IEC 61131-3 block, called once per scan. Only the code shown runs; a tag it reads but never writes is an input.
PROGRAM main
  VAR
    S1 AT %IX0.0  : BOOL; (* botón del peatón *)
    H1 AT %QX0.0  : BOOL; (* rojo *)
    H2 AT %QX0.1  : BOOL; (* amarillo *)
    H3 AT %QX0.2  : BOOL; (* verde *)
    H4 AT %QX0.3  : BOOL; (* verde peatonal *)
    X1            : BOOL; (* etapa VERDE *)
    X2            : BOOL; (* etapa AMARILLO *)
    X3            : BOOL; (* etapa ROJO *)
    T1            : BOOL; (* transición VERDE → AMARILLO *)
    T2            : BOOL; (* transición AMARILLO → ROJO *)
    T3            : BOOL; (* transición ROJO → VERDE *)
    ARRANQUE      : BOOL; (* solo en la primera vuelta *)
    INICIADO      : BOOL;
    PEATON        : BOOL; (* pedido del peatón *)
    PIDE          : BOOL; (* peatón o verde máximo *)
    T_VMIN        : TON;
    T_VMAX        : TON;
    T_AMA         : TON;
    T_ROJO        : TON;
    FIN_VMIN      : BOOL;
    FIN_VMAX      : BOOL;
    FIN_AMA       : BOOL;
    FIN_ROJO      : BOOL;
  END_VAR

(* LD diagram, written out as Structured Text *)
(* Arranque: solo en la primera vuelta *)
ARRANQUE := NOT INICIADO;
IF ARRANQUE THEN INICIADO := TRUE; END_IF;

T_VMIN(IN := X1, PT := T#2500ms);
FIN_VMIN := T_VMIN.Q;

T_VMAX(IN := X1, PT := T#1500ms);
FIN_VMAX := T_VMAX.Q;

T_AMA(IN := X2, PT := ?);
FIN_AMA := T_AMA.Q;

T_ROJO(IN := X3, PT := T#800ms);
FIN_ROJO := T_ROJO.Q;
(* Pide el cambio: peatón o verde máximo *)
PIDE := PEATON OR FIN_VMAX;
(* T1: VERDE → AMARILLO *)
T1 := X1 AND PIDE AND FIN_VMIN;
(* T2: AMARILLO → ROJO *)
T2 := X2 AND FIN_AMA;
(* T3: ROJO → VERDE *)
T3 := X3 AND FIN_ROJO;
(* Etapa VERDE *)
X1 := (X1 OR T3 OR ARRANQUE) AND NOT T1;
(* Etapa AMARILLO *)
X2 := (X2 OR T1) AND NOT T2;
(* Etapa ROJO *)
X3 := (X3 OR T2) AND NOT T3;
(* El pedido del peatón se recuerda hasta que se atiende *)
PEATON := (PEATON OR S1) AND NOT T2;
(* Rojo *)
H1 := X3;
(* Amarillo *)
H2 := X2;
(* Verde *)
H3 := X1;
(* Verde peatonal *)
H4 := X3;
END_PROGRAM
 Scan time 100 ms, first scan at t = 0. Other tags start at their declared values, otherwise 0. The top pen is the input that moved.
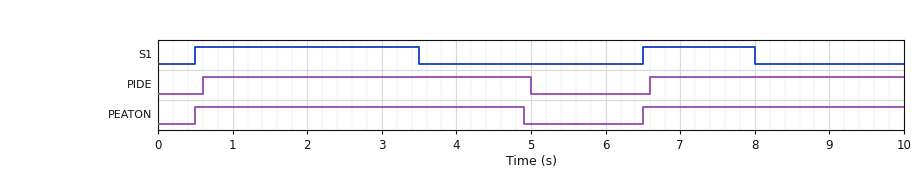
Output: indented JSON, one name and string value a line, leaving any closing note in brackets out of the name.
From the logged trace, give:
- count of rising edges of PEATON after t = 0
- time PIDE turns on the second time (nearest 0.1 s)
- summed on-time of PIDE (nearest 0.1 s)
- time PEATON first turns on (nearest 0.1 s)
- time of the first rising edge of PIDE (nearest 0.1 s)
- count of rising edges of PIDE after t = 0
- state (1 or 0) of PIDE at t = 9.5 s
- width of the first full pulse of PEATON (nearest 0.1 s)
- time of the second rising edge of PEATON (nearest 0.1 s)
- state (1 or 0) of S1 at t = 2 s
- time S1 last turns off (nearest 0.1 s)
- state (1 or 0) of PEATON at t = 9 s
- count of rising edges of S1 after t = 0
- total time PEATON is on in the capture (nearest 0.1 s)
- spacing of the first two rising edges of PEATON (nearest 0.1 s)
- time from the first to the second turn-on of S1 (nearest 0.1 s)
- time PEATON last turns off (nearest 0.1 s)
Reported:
{
  "count of rising edges of PEATON after t = 0": "2",
  "time PIDE turns on the second time": "6.6 s",
  "summed on-time of PIDE": "7.8 s",
  "time PEATON first turns on": "0.5 s",
  "time of the first rising edge of PIDE": "0.6 s",
  "count of rising edges of PIDE after t = 0": "2",
  "state (1 or 0) of PIDE at t = 9.5 s": "1",
  "width of the first full pulse of PEATON": "4.4 s",
  "time of the second rising edge of PEATON": "6.5 s",
  "state (1 or 0) of S1 at t = 2 s": "1",
  "time S1 last turns off": "8.0 s",
  "state (1 or 0) of PEATON at t = 9 s": "1",
  "count of rising edges of S1 after t = 0": "2",
  "total time PEATON is on in the capture": "7.9 s",
  "spacing of the first two rising edges of PEATON": "6.0 s",
  "time from the first to the second turn-on of S1": "6.0 s",
  "time PEATON last turns off": "4.9 s"
}
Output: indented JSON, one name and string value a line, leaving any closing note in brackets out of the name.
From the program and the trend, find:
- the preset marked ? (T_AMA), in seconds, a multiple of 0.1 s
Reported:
{
  "the preset marked ? (T_AMA), in seconds, a multiple of 0.1 s": "2.2 s"
}
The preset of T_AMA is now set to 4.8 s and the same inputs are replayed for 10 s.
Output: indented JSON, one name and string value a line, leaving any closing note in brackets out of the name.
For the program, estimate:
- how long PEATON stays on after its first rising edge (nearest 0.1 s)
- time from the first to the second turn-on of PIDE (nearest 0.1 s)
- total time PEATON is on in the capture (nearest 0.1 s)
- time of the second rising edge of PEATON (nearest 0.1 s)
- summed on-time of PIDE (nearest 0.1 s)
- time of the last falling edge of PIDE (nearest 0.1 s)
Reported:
{
  "how long PEATON stays on after its first rising edge": "7.0 s",
  "time from the first to the second turn-on of PIDE": "7.1 s",
  "total time PEATON is on in the capture": "9.4 s",
  "time of the second rising edge of PEATON": "7.6 s",
  "summed on-time of PIDE": "9.3 s",
  "time of the last falling edge of PIDE": "7.6 s"
}
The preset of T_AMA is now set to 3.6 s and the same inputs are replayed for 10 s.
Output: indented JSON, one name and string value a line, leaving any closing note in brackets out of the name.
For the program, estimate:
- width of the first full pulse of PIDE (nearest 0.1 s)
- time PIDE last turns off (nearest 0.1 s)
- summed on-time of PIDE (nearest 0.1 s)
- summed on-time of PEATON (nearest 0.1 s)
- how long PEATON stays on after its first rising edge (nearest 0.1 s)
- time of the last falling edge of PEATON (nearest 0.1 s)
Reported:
{
  "width of the first full pulse of PIDE": "5.8 s",
  "time PIDE last turns off": "6.4 s",
  "summed on-time of PIDE": "9.2 s",
  "summed on-time of PEATON": "9.3 s",
  "how long PEATON stays on after its first rising edge": "5.8 s",
  "time of the last falling edge of PEATON": "6.3 s"
}
